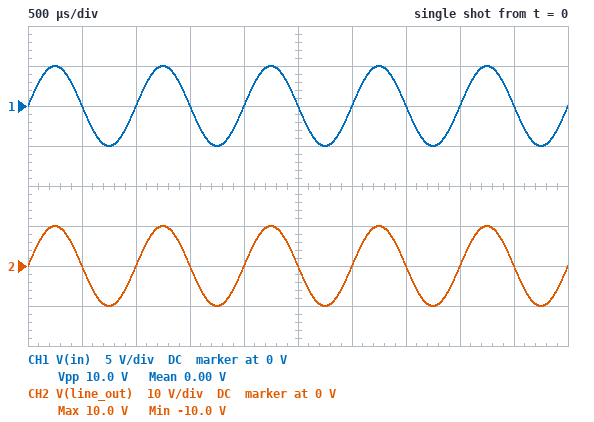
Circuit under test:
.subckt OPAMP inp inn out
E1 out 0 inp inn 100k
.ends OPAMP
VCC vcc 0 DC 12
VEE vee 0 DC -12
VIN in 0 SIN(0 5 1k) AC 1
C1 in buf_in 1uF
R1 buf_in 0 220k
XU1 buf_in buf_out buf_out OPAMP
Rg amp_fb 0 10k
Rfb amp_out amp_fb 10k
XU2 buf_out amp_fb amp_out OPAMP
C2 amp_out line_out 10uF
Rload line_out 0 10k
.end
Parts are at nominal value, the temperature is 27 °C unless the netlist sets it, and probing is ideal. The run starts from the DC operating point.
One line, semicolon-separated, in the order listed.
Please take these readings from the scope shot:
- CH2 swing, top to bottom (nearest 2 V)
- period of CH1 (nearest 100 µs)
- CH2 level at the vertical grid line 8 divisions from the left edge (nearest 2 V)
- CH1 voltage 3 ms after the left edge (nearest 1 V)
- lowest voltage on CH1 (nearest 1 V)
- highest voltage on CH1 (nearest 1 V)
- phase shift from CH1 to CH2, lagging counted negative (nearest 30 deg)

20 V; 1.0 ms; 0 V; 0 V; -5 V; 5 V; 0 deg
